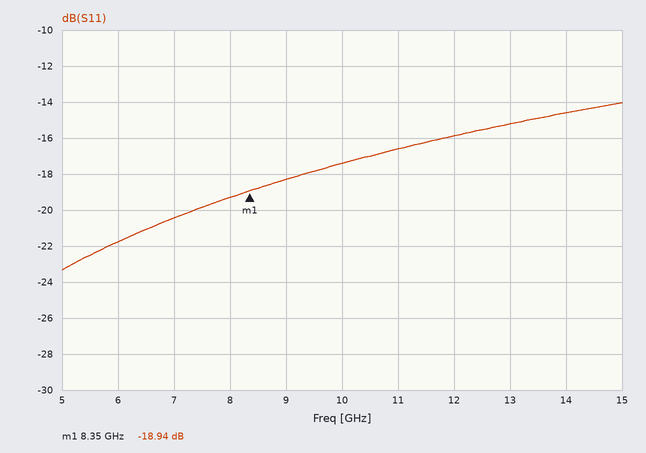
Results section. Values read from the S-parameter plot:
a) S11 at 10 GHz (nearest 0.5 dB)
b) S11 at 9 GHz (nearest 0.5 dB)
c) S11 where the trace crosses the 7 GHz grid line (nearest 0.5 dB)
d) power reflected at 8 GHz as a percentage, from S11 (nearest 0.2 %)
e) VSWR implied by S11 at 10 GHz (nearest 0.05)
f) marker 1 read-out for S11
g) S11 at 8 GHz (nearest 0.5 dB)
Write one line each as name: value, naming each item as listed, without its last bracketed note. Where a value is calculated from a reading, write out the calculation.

S11 at 10 GHz: -17.5 dB
S11 at 9 GHz: -18.5 dB
S11 where the trace crosses the 7 GHz grid line: -20.5 dB
power reflected at 8 GHz as a percentage, from S11: 10^(-19.5/10) ≈ 1.12 %, so 1.2 % to the nearest 0.2 %
VSWR implied by S11 at 10 GHz: |Γ| = 10^(-17.5/20) = 0.1334; VSWR = (1 + 0.1334)/(1 − 0.1334) ≈ 1.31, so 1.30 to the nearest 0.05
marker 1 read-out for S11: -18.94 dB
S11 at 8 GHz: -19.5 dB
